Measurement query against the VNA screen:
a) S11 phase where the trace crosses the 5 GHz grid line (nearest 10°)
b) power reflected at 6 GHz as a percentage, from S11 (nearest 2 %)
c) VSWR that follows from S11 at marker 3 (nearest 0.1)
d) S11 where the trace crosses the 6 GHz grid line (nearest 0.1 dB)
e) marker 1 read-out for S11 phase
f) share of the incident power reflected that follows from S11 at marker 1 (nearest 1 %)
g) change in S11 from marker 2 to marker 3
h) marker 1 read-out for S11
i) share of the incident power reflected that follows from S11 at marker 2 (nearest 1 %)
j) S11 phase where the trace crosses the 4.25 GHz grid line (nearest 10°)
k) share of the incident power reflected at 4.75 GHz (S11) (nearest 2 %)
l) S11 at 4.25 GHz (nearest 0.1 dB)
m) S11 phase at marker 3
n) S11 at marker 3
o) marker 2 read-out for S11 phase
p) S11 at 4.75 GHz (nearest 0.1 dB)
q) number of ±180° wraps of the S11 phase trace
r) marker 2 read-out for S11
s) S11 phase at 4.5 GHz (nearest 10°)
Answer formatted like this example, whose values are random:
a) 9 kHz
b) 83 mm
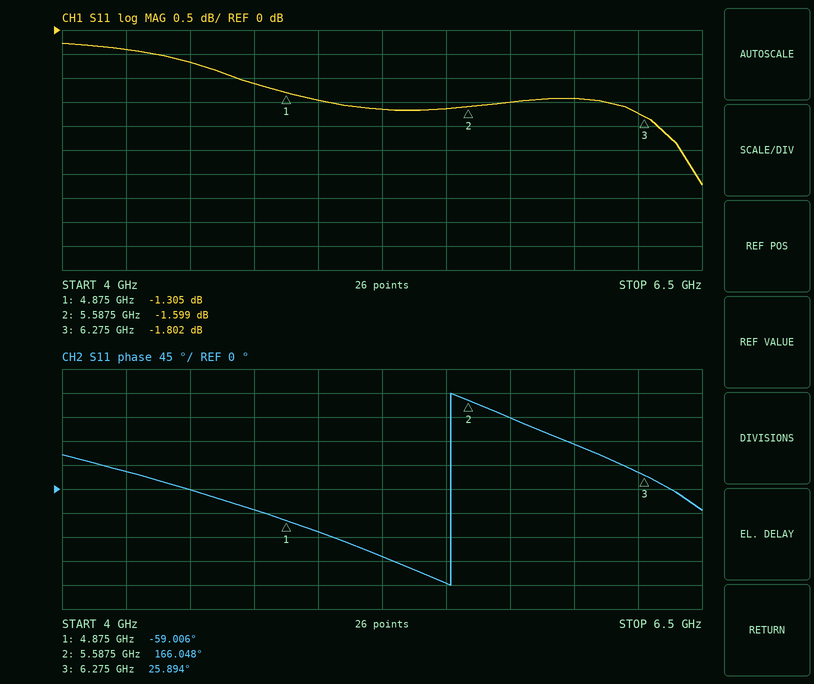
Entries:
a) -80°
b) 72 %
c) 9.7
d) -1.4 dB
e) -59.006°
f) 74 %
g) -0.203 dB
h) -1.305 dB
i) 69 %
j) 30°
k) 78 %
l) -0.4 dB
m) 25.894°
n) -1.802 dB
o) 166.048°
p) -1.1 dB
q) 1
r) -1.599 dB
s) 0°
